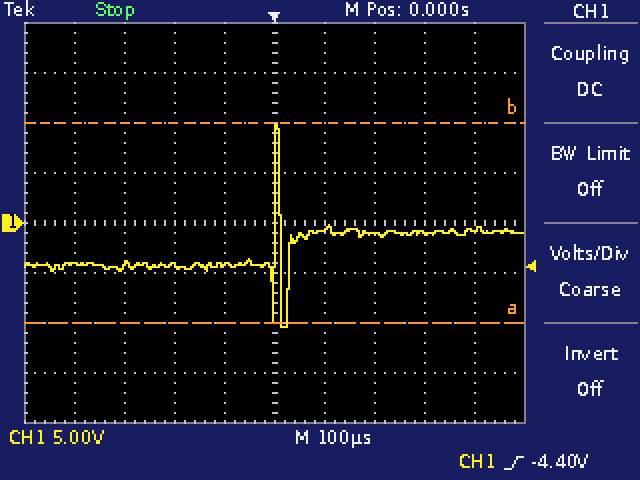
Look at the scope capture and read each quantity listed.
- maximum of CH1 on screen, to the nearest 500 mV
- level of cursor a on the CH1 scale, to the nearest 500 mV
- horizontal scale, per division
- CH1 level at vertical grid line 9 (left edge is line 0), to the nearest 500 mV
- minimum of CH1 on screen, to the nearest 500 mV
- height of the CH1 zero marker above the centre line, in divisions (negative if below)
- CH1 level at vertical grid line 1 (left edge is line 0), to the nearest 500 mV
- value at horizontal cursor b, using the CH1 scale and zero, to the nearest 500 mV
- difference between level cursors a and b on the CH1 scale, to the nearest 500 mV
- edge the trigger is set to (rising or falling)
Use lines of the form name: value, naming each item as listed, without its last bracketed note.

maximum of CH1 on screen, to the nearest 500 mV: 10.0 V
level of cursor a on the CH1 scale, to the nearest 500 mV: -10.0 V
horizontal scale, per division: 100 µs
CH1 level at vertical grid line 9 (left edge is line 0), to the nearest 500 mV: -500 mV
minimum of CH1 on screen, to the nearest 500 mV: -10.5 V
height of the CH1 zero marker above the centre line, in divisions: 0.0 div
CH1 level at vertical grid line 1 (left edge is line 0), to the nearest 500 mV: -4.0 V
value at horizontal cursor b, using the CH1 scale and zero, to the nearest 500 mV: 10.0 V
difference between level cursors a and b on the CH1 scale, to the nearest 500 mV: 20.0 V
edge the trigger is set to: rising
